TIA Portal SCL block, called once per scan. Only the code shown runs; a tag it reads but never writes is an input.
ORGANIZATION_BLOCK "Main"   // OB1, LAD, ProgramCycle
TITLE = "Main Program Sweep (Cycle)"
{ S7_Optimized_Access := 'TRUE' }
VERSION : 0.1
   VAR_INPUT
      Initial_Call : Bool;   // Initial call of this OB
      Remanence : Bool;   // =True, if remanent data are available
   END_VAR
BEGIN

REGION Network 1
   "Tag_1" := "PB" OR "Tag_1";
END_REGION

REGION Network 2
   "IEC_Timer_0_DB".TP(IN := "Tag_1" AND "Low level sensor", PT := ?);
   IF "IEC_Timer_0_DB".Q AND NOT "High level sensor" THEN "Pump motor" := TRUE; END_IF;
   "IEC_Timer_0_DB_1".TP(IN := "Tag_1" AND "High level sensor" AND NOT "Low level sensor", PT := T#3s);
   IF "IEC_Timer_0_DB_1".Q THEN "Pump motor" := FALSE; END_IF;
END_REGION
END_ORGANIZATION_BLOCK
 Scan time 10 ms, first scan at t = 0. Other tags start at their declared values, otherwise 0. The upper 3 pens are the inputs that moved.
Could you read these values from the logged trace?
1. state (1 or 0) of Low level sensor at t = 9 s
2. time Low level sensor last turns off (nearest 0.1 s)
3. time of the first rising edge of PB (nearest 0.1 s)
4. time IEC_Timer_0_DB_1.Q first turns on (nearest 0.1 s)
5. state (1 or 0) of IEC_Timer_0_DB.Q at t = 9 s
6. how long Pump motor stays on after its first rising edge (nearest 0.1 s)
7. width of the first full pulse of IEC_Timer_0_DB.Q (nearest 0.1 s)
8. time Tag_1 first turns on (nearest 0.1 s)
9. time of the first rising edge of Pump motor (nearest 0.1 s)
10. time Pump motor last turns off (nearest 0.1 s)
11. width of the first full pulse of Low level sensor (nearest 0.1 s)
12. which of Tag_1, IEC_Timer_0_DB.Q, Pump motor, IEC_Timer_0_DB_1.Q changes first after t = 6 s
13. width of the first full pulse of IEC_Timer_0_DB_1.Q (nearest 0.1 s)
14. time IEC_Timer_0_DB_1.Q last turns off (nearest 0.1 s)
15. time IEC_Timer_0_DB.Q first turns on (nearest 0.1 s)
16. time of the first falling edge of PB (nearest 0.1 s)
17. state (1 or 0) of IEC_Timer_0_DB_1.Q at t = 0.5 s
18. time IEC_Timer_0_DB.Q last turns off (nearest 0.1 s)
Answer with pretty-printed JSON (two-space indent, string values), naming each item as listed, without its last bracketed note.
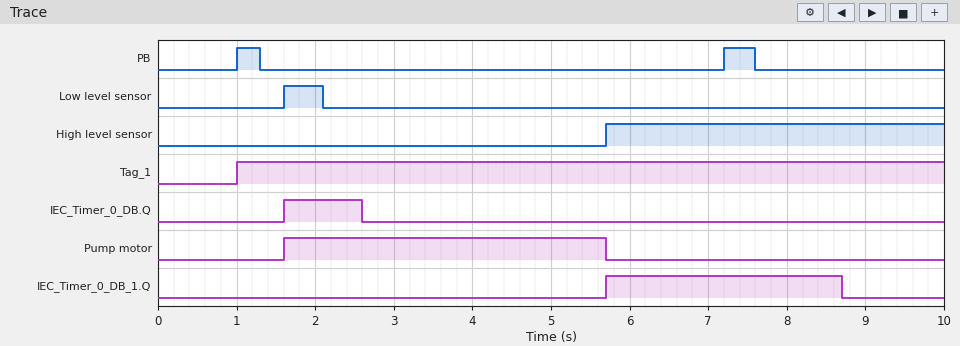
{
  "state (1 or 0) of Low level sensor at t = 9 s": "0",
  "time Low level sensor last turns off": "2.1 s",
  "time of the first rising edge of PB": "1.0 s",
  "time IEC_Timer_0_DB_1.Q first turns on": "5.7 s",
  "state (1 or 0) of IEC_Timer_0_DB.Q at t = 9 s": "0",
  "how long Pump motor stays on after its first rising edge": "4.1 s",
  "width of the first full pulse of IEC_Timer_0_DB.Q": "1.0 s",
  "time Tag_1 first turns on": "1.0 s",
  "time of the first rising edge of Pump motor": "1.6 s",
  "time Pump motor last turns off": "5.7 s",
  "width of the first full pulse of Low level sensor": "0.5 s",
  "which of Tag_1, IEC_Timer_0_DB.Q, Pump motor, IEC_Timer_0_DB_1.Q changes first after t = 6 s": "IEC_Timer_0_DB_1.Q",
  "width of the first full pulse of IEC_Timer_0_DB_1.Q": "3.0 s",
  "time IEC_Timer_0_DB_1.Q last turns off": "8.7 s",
  "time IEC_Timer_0_DB.Q first turns on": "1.6 s",
  "time of the first falling edge of PB": "1.3 s",
  "state (1 or 0) of IEC_Timer_0_DB_1.Q at t = 0.5 s": "0",
  "time IEC_Timer_0_DB.Q last turns off": "2.6 s"
}
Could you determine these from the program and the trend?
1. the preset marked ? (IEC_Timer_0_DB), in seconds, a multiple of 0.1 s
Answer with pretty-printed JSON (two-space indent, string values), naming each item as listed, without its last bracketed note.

{
  "the preset marked ? (IEC_Timer_0_DB), in seconds, a multiple of 0.1 s": "1.0 s"
}
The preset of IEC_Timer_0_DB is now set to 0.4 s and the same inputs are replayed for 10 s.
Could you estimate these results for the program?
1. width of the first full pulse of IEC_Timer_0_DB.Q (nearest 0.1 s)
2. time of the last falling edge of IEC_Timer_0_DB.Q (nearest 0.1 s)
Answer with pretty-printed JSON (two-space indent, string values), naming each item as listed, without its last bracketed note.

{
  "width of the first full pulse of IEC_Timer_0_DB.Q": "0.4 s",
  "time of the last falling edge of IEC_Timer_0_DB.Q": "2.0 s"
}
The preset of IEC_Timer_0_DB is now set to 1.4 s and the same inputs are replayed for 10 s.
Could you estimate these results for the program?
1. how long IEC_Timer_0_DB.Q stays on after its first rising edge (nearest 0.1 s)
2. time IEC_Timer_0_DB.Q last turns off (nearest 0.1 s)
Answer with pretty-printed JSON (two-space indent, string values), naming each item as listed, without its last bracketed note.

{
  "how long IEC_Timer_0_DB.Q stays on after its first rising edge": "1.4 s",
  "time IEC_Timer_0_DB.Q last turns off": "3.0 s"
}
